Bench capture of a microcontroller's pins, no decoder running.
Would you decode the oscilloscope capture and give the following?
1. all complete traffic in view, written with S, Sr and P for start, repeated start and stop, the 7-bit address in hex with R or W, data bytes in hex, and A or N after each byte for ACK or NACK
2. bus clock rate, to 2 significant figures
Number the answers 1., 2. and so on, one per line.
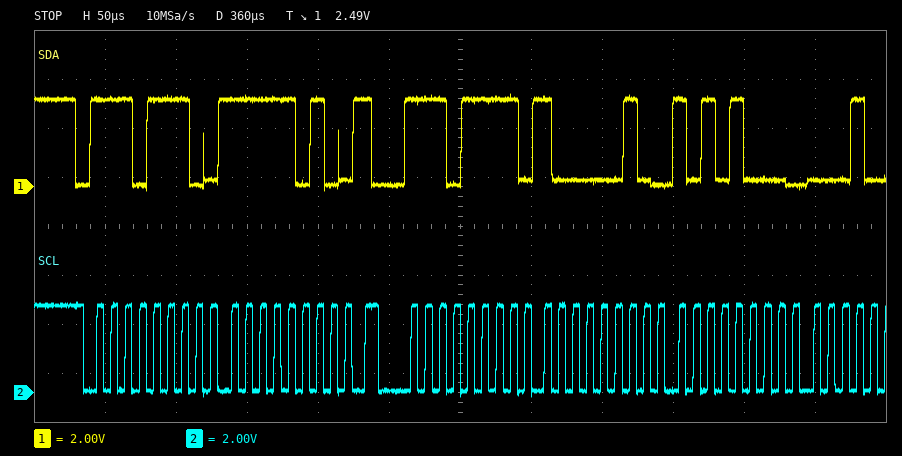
1. S 77W A FA A Sr 77R A 82 A A8 A
2. 100 kHz
